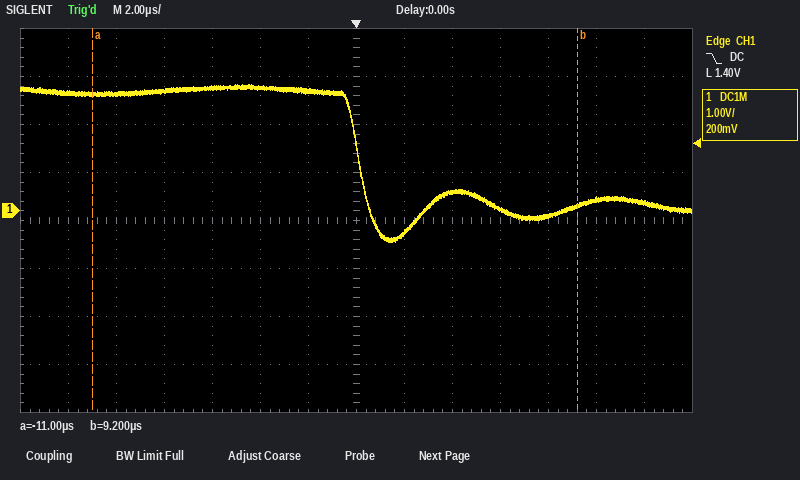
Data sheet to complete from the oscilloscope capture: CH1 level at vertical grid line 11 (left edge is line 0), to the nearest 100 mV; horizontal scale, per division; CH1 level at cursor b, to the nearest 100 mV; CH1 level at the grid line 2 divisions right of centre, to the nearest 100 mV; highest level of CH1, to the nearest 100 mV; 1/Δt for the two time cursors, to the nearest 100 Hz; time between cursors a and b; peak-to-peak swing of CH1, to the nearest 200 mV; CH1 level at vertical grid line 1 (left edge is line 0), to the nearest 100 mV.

-100 mV
2 µs
100 mV
400 mV
2.6 V
49.5 kHz
20.2 µs
3.2 V
2.5 V
